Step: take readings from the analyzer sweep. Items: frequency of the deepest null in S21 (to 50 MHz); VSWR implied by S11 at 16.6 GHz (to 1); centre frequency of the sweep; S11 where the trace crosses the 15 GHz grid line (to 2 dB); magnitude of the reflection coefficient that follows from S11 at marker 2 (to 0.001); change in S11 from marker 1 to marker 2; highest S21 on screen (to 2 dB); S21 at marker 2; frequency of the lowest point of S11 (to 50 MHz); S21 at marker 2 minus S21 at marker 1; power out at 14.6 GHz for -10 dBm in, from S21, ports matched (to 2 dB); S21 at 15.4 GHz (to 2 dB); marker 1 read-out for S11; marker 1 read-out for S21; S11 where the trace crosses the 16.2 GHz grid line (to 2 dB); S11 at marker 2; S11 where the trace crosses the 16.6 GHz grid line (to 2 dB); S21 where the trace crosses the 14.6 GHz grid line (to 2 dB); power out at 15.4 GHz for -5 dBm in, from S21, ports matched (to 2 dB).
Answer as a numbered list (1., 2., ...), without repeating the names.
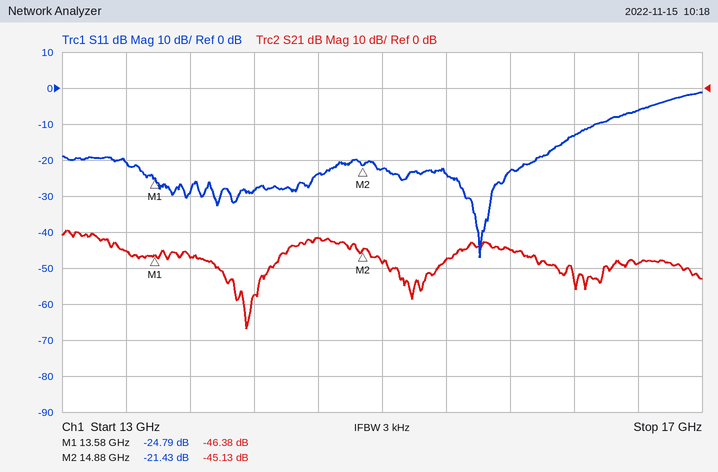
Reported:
1. 14.15 GHz
2. 3
3. 15 GHz
4. -22 dB
5. 0.085
6. 3.36 dB
7. -40 dB
8. -45.13 dB
9. 15.60 GHz
10. 1.25 dB
11. -52 dBm
12. -48 dB
13. -24.79 dB
14. -46.38 dB
15. -14 dB
16. -21.43 dB
17. -6 dB
18. -42 dB
19. -52 dBm
